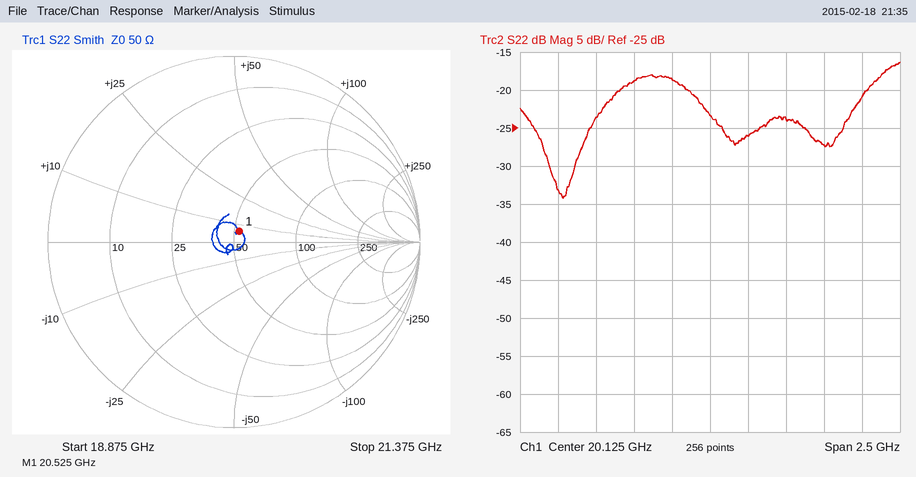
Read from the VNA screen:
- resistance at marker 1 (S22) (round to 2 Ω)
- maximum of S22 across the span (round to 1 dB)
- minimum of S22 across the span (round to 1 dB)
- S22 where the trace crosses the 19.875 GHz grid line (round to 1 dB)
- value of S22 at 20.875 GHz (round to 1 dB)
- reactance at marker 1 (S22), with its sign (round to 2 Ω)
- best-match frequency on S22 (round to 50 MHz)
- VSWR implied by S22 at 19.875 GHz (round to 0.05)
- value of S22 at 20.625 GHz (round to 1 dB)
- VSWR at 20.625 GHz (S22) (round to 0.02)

52 Ω
-16 dB
-34 dB
-19 dB
-27 dB
+6 Ω
19.15 GHz
1.25
-24 dB
1.14
